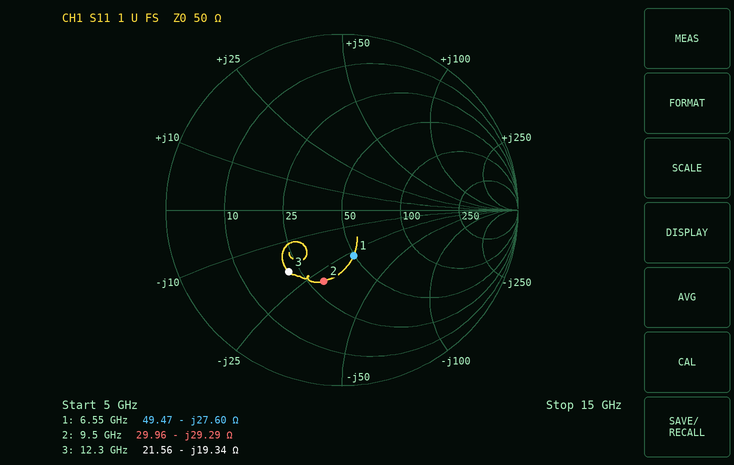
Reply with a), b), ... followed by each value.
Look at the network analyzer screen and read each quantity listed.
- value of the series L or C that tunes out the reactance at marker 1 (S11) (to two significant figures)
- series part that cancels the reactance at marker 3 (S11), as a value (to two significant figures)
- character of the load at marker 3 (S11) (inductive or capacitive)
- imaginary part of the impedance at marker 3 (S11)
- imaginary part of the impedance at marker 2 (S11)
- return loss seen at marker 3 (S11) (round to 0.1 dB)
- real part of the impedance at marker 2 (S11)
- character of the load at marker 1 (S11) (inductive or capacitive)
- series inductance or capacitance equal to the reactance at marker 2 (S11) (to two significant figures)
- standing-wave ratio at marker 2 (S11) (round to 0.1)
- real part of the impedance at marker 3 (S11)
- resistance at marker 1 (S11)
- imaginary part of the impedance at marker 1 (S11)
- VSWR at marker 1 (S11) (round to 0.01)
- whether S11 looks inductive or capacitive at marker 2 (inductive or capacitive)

a) 670 pH
b) 250 pH
c) capacitive
d) -19.34 Ω
e) -29.29 Ω
f) 6.7 dB
g) 29.96 Ω
h) capacitive
i) 570 fF
j) 2.4
k) 21.56 Ω
l) 49.47 Ω
m) -27.60 Ω
n) 1.73
o) capacitive
